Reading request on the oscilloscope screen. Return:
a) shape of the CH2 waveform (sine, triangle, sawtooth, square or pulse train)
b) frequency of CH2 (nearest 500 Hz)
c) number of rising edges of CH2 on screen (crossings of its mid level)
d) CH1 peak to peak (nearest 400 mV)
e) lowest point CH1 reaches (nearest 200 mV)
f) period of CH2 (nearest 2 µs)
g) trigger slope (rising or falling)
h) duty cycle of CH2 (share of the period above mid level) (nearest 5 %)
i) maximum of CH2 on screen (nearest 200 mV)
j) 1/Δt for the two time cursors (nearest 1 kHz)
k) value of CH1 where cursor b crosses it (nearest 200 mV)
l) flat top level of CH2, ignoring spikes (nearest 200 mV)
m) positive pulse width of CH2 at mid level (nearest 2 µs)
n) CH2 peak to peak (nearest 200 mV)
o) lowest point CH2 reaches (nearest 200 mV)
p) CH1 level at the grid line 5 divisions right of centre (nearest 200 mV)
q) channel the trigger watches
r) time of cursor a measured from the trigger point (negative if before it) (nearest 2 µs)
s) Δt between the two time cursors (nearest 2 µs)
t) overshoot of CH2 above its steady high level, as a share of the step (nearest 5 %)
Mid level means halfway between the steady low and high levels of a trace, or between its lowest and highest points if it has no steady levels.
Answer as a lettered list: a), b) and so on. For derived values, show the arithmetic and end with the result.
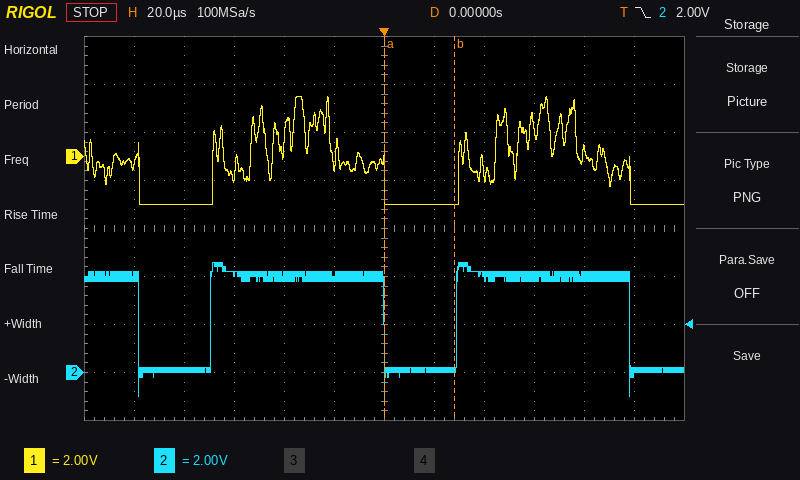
a) pulse train
b) 1 / 98 µs ≈ 10.2 kHz, so 10.0 kHz to the nearest 500 Hz
c) 2
d) 4.4 V
e) -2.0 V
f) 98 µs
g) falling
h) 70 µs / 98 µs ≈ 71.4 %, so 70 % to the nearest 5 %
i) 4.6 V
j) 1 / 28 µs ≈ 36 kHz
k) -2.0 V
l) 4.0 V
m) 70 µs
n) 4.6 V − (-1.0 V) = 5.6 V
o) -1.0 V
p) -2.0 V
q) CH2
r) 0 µs
s) 28 µs
t) 15 %
